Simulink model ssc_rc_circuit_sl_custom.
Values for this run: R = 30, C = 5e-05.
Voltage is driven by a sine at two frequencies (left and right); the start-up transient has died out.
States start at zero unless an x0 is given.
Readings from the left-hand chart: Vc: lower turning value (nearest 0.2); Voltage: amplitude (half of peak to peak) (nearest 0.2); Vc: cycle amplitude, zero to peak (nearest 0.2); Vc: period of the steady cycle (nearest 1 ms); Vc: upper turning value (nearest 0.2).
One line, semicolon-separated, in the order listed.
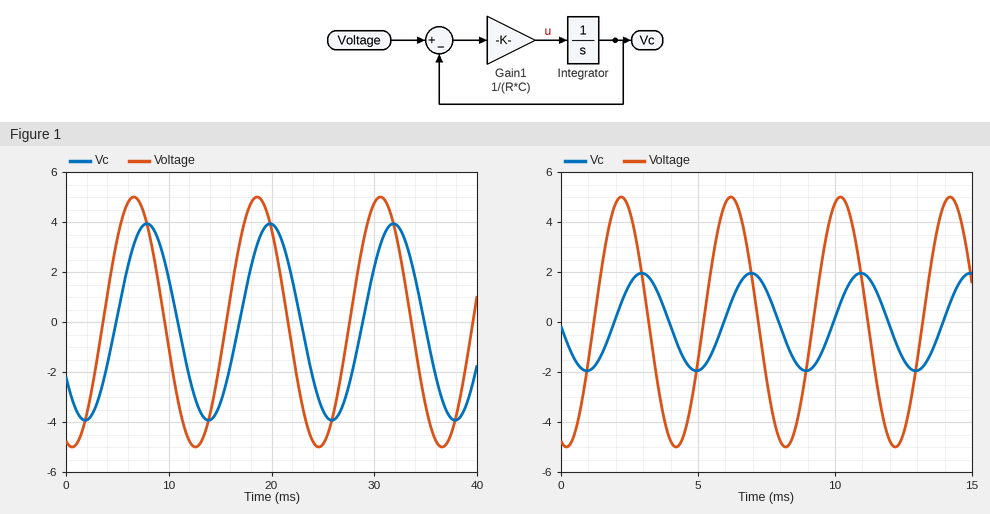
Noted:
-4.0; 5.0; 4.0; 12 ms; 4.0
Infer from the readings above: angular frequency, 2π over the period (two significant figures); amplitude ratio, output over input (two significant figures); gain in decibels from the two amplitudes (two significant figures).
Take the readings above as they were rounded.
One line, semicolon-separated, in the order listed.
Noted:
0.52 rad/ms; 0.80; -1.9 dB
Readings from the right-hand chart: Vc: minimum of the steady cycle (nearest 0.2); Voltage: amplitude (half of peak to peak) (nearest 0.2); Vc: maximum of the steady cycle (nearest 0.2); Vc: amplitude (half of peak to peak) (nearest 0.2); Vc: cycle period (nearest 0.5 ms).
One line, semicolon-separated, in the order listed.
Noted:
-2.0; 5.0; 2.0; 2.0; 4.0 ms
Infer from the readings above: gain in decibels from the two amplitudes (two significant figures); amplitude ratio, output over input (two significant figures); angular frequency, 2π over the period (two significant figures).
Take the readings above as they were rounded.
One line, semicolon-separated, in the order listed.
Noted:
-8.0 dB; 0.40; 1.6 rad/ms
